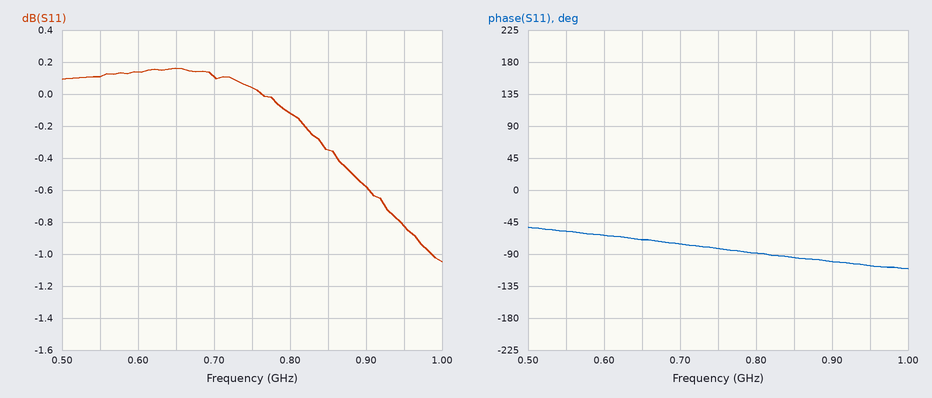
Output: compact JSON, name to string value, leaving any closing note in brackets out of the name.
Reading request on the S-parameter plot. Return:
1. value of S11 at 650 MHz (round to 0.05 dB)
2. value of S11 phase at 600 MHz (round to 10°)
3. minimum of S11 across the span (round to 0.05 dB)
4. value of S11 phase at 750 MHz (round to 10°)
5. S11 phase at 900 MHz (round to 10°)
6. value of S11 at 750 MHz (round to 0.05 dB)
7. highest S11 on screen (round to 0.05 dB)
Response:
{"value of S11 at 650 MHz": "0.15 dB", "value of S11 phase at 600 MHz": "-60°", "minimum of S11 across the span": "-1.05 dB", "value of S11 phase at 750 MHz": "-80°", "S11 phase at 900 MHz": "-100°", "value of S11 at 750 MHz": "0.05 dB", "highest S11 on screen": "0.15 dB"}
